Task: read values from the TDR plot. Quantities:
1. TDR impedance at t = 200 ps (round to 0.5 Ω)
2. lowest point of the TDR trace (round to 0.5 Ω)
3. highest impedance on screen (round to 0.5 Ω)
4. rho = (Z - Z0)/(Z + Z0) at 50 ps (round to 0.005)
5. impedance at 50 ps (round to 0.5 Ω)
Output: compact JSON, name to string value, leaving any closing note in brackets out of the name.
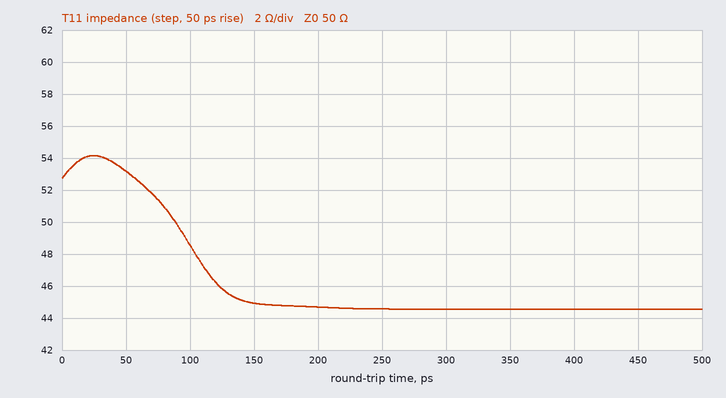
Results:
{"TDR impedance at t = 200 ps": "44.5 Ω", "lowest point of the TDR trace": "44.5 Ω", "highest impedance on screen": "54.0 Ω", "rho = (Z - Z0)/(Z + Z0) at 50 ps": "+0.030", "impedance at 50 ps": "53.0 Ω"}
